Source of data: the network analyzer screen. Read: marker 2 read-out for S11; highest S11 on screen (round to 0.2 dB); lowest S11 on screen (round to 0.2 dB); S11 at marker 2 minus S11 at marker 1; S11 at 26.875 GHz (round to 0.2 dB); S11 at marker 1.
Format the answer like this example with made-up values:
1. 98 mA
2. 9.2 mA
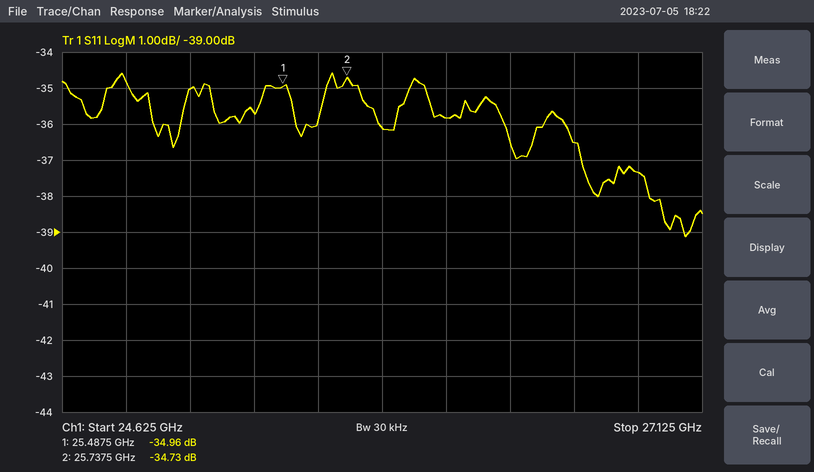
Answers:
1. -34.73 dB
2. -34.6 dB
3. -39.2 dB
4. 0.23 dB
5. -37.4 dB
6. -34.96 dB
